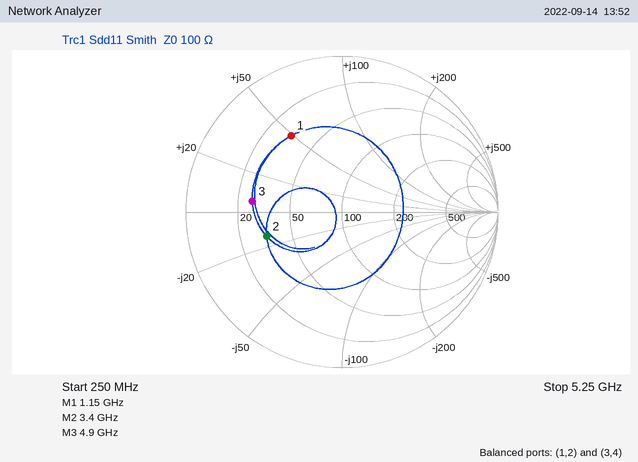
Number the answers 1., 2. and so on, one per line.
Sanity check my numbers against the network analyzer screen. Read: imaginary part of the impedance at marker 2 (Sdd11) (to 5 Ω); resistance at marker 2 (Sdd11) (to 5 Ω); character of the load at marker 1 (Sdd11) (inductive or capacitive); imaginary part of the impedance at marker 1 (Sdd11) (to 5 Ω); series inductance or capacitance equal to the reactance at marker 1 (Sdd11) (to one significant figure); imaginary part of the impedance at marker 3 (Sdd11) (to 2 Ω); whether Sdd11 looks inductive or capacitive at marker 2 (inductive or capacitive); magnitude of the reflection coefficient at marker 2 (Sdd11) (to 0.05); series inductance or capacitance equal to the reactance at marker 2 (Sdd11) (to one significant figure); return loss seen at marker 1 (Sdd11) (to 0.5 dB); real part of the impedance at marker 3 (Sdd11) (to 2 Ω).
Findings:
1. -15 Ω
2. 35 Ω
3. inductive
4. +50 Ω
5. 7 nH
6. +6 Ω
7. capacitive
8. 0.50
9. 3 pF
10. 4.5 dB
11. 26 Ω
